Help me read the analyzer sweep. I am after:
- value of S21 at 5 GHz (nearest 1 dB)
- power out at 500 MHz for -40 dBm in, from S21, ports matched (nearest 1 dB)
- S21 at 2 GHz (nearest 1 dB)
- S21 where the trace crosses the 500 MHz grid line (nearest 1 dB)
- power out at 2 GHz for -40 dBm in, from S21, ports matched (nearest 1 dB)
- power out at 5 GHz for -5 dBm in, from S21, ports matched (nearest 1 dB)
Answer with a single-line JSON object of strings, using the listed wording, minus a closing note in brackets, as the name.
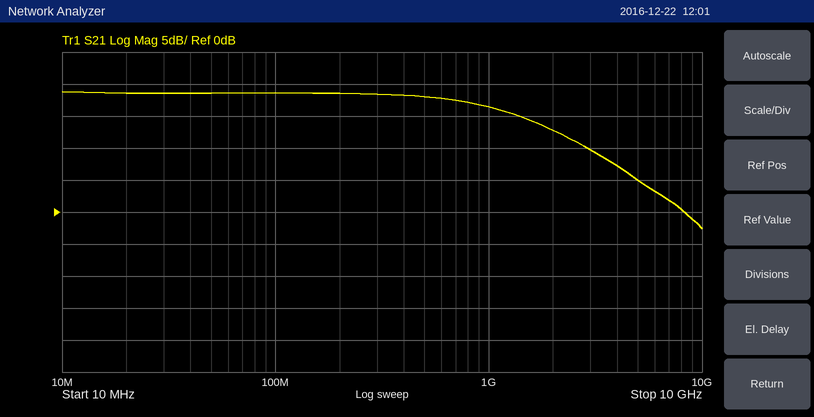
{"value of S21 at 5 GHz": "5 dB", "power out at 500 MHz for -40 dBm in, from S21, ports matched": "-22 dBm", "S21 at 2 GHz": "13 dB", "S21 where the trace crosses the 500 MHz grid line": "18 dB", "power out at 2 GHz for -40 dBm in, from S21, ports matched": "-27 dBm", "power out at 5 GHz for -5 dBm in, from S21, ports matched": "0 dBm"}
